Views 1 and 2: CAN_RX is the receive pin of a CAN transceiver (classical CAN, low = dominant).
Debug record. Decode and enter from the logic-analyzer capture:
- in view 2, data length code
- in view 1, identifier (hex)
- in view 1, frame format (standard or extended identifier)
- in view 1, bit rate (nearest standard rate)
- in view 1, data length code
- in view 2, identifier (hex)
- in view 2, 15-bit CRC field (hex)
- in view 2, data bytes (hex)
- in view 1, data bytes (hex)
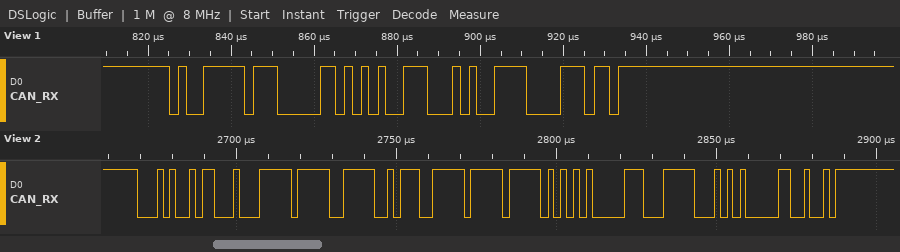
8
0x4FF
standard
500 kbit/s
2
0x14B
0x2824
FF DF 5C FF FF 54 18 F9
A9 C5
